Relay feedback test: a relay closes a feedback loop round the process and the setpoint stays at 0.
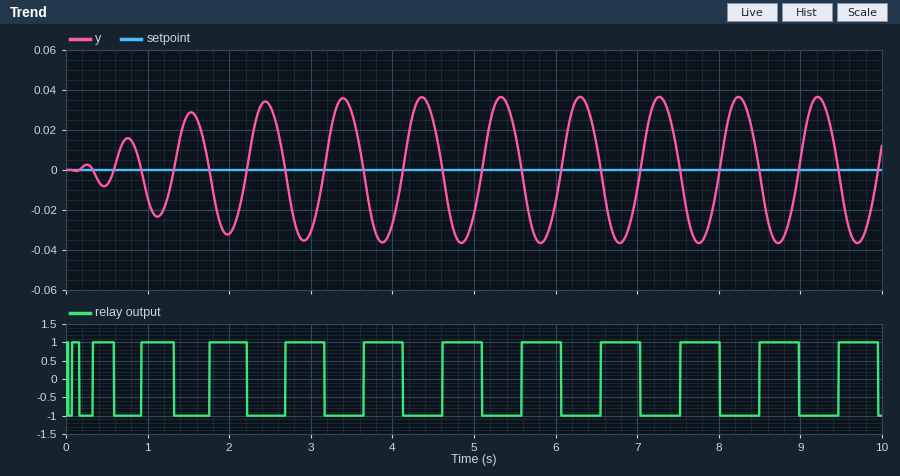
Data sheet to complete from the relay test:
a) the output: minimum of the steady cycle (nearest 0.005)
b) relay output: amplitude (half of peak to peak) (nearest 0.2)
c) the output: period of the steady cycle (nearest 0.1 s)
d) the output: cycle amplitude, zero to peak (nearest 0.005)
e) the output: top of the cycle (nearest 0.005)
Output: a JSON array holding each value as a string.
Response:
["-0.035", "1.0", "1.0 s", "0.035", "0.035"]
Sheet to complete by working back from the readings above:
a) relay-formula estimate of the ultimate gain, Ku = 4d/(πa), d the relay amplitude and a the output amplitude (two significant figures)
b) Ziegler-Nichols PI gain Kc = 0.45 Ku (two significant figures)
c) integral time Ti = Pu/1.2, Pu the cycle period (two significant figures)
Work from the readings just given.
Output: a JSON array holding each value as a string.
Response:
["36", "16", "0.83 s"]
